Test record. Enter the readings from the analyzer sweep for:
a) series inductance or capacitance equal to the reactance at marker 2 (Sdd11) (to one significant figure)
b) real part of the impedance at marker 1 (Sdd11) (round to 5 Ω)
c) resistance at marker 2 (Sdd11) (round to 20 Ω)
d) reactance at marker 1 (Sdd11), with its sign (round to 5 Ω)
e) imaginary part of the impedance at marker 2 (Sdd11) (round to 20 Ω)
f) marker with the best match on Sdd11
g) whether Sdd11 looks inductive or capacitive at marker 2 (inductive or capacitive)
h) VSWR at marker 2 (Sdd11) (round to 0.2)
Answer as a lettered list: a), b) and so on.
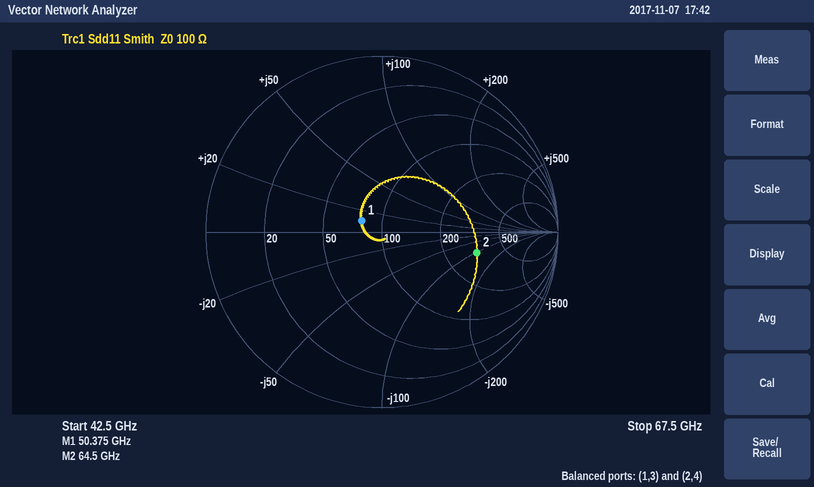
a) 20 fF
b) 80 Ω
c) 300 Ω
d) +10 Ω
e) -100 Ω
f) marker 1
g) capacitive
h) 3.4
